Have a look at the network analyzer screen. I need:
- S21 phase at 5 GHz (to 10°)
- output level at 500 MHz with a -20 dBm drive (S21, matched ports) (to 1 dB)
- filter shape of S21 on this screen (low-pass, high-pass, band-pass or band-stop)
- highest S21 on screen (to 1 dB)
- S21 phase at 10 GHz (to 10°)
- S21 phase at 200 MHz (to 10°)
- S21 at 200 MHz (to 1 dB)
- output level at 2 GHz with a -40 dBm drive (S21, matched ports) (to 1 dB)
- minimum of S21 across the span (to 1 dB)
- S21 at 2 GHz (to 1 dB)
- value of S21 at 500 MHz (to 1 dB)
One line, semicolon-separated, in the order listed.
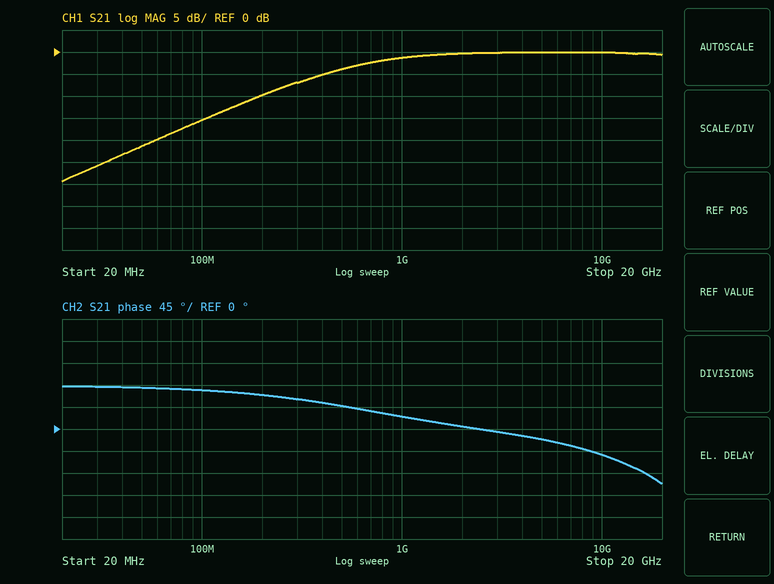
-20°; -24 dBm; high-pass; 0 dB; -50°; 70°; -10 dB; -40 dBm; -29 dB; 0 dB; -4 dB
